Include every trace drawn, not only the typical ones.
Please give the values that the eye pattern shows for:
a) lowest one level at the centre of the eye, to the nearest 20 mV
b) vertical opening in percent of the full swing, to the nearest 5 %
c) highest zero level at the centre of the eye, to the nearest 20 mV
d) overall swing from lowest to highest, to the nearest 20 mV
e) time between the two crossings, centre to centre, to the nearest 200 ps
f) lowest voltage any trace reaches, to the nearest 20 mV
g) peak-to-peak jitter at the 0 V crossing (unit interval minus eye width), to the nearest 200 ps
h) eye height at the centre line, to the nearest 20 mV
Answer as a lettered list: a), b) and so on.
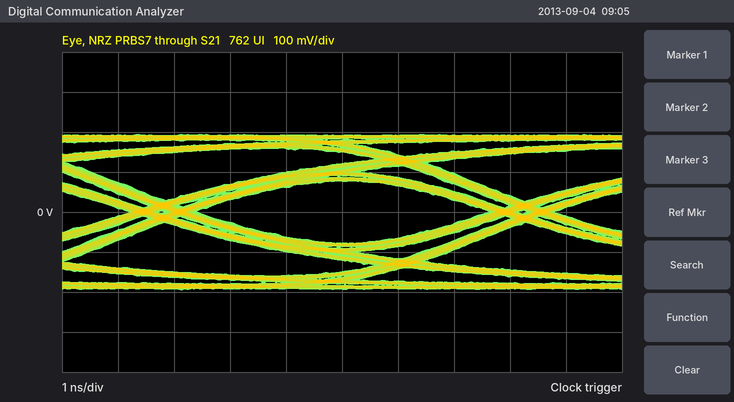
a) 80 mV
b) 40 %
c) -80 mV
d) 380 mV
e) 6.4 ns
f) -200 mV
g) 1.2 ns
h) 160 mV
